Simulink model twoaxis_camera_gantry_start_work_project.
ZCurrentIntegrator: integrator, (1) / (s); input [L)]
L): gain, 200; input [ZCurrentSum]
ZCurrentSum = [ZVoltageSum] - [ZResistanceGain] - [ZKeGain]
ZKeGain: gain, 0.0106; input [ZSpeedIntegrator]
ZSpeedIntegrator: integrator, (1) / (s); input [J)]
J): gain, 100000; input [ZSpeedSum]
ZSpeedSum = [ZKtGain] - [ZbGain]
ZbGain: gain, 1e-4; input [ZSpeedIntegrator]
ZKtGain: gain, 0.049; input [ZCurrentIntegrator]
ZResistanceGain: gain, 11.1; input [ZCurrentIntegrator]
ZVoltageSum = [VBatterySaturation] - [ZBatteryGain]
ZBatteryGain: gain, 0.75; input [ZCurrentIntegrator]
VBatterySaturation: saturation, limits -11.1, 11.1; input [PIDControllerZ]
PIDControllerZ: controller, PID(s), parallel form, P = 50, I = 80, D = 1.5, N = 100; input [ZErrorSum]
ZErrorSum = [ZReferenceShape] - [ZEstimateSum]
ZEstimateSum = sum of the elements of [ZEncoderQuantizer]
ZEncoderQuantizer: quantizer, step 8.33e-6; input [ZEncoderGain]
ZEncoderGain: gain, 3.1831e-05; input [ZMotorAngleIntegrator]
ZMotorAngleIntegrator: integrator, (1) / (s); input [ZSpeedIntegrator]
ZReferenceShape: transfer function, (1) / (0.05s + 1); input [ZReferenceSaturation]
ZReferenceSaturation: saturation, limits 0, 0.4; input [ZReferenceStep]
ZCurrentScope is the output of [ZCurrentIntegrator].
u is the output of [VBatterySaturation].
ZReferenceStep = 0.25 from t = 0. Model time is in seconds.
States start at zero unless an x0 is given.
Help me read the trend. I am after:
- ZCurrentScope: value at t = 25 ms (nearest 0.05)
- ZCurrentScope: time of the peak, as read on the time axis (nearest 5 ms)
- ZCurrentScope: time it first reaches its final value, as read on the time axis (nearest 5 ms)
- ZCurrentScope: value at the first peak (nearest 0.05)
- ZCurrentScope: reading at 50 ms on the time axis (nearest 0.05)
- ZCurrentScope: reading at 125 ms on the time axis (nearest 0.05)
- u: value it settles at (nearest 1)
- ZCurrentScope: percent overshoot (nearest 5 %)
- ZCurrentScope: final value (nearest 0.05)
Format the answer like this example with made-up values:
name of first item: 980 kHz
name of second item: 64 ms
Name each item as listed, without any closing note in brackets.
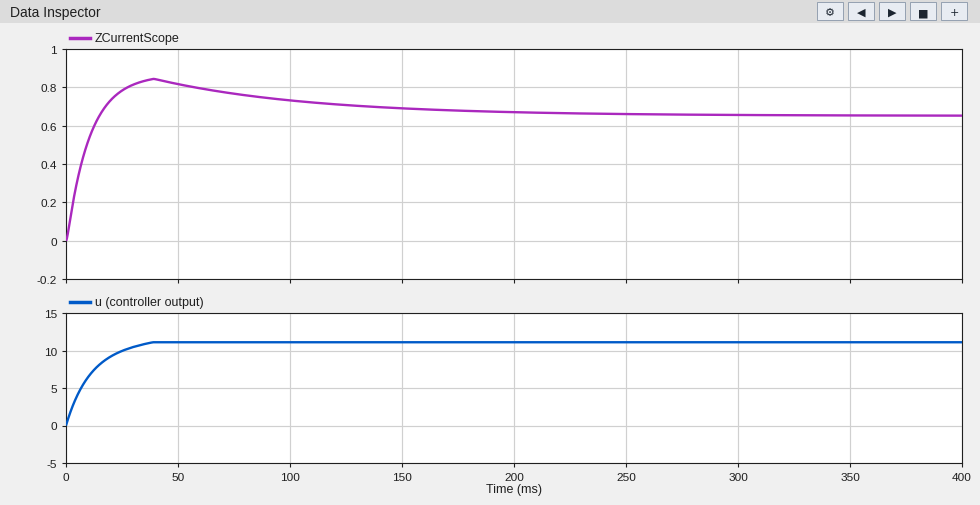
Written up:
ZCurrentScope: value at t = 25 ms: 0.80
ZCurrentScope: time of the peak, as read on the time axis: 40 ms
ZCurrentScope: time it first reaches its final value, as read on the time axis: 15 ms
ZCurrentScope: value at the first peak: 0.85
ZCurrentScope: reading at 50 ms on the time axis: 0.80
ZCurrentScope: reading at 125 ms on the time axis: 0.70
u: value it settles at: 11
ZCurrentScope: percent overshoot: 30 %
ZCurrentScope: final value: 0.65
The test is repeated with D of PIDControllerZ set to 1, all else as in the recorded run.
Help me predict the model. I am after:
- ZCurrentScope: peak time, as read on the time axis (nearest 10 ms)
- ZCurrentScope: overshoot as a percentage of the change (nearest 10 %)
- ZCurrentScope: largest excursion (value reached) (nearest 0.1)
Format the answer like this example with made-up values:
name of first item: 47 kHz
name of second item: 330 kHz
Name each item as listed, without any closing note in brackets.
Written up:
ZCurrentScope: peak time, as read on the time axis: 60 ms
ZCurrentScope: overshoot as a percentage of the change: 20 %
ZCurrentScope: largest excursion (value reached): 0.8
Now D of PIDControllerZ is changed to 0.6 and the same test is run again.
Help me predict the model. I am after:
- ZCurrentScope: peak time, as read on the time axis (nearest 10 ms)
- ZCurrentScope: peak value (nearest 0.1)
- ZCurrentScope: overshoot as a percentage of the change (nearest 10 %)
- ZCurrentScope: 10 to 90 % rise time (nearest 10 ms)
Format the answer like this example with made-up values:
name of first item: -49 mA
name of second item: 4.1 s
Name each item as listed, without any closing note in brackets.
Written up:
ZCurrentScope: peak time, as read on the time axis: 70 ms
ZCurrentScope: peak value: 0.8
ZCurrentScope: overshoot as a percentage of the change: 20 %
ZCurrentScope: 10 to 90 % rise time: 30 ms
